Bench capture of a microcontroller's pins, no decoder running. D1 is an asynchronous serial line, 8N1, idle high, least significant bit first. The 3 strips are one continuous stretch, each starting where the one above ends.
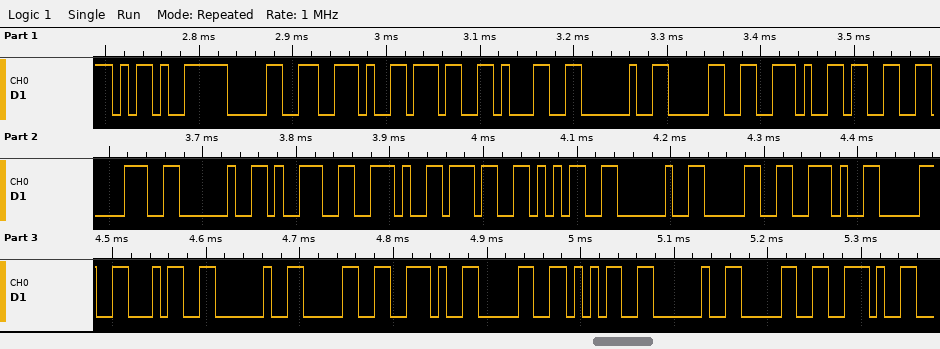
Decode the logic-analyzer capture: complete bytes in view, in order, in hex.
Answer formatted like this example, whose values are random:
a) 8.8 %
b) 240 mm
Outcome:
a) 0x2D 0x30 0x2E 0x37 0x31 0x20 0x30 0x2E 0x33 0x38 0x20 0x39 0x2E 0x37 0x35 0x20 0x30 0x2E 0x30 0x34 0x20 0x30 0x2E 0x30 0x35 0x20 0x30 0x2E
